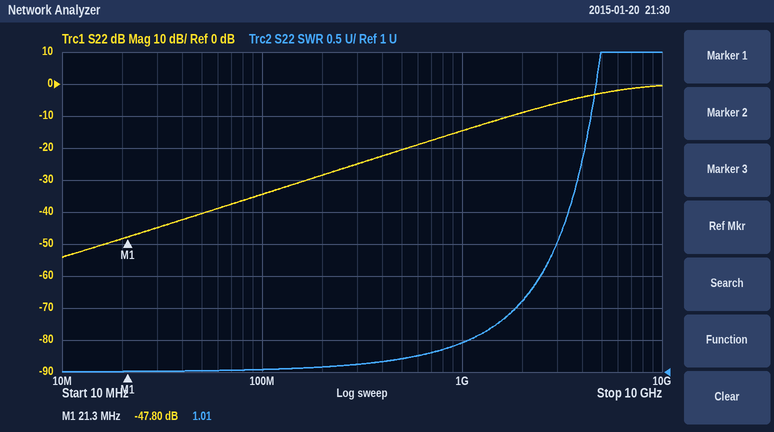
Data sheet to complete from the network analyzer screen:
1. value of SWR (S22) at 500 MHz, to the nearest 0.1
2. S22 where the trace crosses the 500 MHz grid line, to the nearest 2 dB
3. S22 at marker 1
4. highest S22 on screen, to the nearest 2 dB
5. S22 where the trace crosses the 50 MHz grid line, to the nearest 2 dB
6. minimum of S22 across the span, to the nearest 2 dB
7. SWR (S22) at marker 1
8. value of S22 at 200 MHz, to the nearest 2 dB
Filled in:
1.2
-20 dB
-47.80 dB
0 dB
-40 dB
-54 dB
1.01
-28 dB
